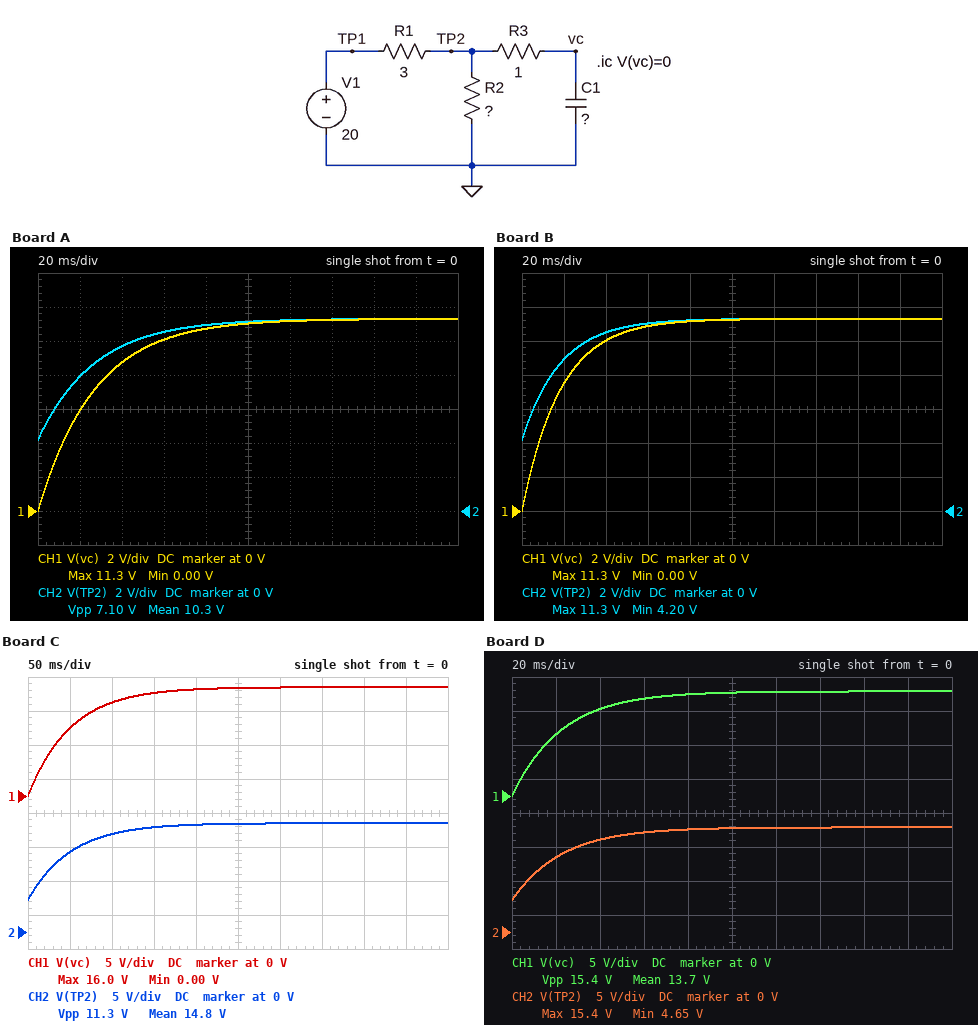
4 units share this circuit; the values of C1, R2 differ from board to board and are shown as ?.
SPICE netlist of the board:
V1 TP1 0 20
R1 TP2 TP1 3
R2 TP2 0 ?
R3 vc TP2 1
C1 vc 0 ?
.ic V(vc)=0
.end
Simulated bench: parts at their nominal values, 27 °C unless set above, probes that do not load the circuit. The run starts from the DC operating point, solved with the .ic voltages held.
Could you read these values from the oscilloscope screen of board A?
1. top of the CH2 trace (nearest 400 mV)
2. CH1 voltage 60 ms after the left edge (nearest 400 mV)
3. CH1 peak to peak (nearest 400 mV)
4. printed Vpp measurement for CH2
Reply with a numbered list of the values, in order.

1. 11.2 V
2. 10.0 V
3. 11.2 V
4. 7.10 V
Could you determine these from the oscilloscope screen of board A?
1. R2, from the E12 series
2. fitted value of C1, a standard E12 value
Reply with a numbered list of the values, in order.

1. 3.9 Ω
2. 10 mF
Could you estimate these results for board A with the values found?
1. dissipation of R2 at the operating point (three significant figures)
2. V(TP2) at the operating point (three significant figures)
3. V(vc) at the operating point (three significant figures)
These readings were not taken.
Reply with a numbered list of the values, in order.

1. 32.8 W
2. 11.3 V
3. 11.3 V
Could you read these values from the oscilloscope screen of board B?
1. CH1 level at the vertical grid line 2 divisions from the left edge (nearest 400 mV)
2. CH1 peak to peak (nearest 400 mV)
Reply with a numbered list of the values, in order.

1. 10.0 V
2. 11.2 V
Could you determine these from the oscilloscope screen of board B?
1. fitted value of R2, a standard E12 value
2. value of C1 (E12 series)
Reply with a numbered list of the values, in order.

1. 3.9 Ω
2. 6.8 mF
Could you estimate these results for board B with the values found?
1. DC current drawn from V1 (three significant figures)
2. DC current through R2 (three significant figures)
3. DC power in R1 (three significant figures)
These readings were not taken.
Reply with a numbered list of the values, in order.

1. 2.90 A
2. 2.90 A
3. 25.2 W
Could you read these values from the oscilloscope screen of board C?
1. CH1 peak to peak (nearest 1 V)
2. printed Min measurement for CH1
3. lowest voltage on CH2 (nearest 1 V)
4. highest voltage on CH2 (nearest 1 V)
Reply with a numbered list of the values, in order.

1. 16 V
2. 0.00 V
3. 5 V
4. 16 V
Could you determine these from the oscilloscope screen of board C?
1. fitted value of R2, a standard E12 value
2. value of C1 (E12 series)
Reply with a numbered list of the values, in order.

1. 12 Ω
2. 15 mF
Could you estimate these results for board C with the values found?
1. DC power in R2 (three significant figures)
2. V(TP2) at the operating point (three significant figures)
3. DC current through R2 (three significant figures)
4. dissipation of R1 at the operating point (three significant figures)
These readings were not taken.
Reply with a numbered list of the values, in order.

1. 21.3 W
2. 16.0 V
3. 1.33 A
4. 5.33 W
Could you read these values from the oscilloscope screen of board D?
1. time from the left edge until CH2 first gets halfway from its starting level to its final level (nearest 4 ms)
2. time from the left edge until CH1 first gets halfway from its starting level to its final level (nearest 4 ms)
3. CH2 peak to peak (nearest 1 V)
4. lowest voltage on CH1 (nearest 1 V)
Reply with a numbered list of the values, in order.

1. 16 ms
2. 16 ms
3. 11 V
4. 0 V
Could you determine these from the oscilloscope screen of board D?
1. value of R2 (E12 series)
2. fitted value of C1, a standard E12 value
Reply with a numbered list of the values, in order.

1. 10 Ω
2. 6.8 mF
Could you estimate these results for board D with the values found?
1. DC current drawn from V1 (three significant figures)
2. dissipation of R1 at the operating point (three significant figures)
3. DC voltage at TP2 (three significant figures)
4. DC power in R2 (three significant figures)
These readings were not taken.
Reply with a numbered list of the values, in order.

1. 1.54 A
2. 7.10 W
3. 15.4 V
4. 23.7 W
